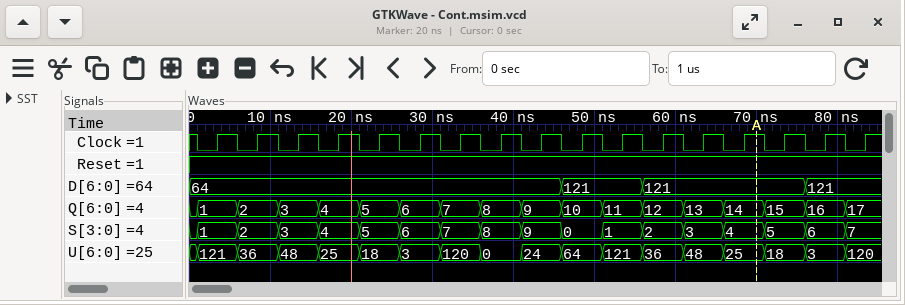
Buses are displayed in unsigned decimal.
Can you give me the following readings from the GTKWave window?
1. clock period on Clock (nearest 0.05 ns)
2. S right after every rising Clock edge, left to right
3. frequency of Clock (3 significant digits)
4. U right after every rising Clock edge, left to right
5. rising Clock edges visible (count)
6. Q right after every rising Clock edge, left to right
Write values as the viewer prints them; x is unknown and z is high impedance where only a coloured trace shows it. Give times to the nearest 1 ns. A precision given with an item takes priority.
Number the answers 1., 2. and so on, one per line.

1. 5 ns
2. 1, 2, 3, 4, 5, 6, 7, 8, 9, 0, 1, 2, 3, 4, 5, 6, 7
3. 200 MHz
4. 121, 36, 48, 25, 18, 3, 120, 0, 24, 64, 121, 36, 48, 25, 18, 3, 120
5. 17
6. 1, 2, 3, 4, 5, 6, 7, 8, 9, 10, 11, 12, 13, 14, 15, 16, 17
